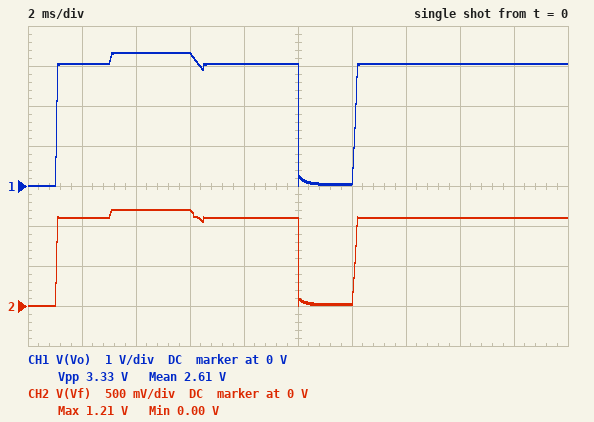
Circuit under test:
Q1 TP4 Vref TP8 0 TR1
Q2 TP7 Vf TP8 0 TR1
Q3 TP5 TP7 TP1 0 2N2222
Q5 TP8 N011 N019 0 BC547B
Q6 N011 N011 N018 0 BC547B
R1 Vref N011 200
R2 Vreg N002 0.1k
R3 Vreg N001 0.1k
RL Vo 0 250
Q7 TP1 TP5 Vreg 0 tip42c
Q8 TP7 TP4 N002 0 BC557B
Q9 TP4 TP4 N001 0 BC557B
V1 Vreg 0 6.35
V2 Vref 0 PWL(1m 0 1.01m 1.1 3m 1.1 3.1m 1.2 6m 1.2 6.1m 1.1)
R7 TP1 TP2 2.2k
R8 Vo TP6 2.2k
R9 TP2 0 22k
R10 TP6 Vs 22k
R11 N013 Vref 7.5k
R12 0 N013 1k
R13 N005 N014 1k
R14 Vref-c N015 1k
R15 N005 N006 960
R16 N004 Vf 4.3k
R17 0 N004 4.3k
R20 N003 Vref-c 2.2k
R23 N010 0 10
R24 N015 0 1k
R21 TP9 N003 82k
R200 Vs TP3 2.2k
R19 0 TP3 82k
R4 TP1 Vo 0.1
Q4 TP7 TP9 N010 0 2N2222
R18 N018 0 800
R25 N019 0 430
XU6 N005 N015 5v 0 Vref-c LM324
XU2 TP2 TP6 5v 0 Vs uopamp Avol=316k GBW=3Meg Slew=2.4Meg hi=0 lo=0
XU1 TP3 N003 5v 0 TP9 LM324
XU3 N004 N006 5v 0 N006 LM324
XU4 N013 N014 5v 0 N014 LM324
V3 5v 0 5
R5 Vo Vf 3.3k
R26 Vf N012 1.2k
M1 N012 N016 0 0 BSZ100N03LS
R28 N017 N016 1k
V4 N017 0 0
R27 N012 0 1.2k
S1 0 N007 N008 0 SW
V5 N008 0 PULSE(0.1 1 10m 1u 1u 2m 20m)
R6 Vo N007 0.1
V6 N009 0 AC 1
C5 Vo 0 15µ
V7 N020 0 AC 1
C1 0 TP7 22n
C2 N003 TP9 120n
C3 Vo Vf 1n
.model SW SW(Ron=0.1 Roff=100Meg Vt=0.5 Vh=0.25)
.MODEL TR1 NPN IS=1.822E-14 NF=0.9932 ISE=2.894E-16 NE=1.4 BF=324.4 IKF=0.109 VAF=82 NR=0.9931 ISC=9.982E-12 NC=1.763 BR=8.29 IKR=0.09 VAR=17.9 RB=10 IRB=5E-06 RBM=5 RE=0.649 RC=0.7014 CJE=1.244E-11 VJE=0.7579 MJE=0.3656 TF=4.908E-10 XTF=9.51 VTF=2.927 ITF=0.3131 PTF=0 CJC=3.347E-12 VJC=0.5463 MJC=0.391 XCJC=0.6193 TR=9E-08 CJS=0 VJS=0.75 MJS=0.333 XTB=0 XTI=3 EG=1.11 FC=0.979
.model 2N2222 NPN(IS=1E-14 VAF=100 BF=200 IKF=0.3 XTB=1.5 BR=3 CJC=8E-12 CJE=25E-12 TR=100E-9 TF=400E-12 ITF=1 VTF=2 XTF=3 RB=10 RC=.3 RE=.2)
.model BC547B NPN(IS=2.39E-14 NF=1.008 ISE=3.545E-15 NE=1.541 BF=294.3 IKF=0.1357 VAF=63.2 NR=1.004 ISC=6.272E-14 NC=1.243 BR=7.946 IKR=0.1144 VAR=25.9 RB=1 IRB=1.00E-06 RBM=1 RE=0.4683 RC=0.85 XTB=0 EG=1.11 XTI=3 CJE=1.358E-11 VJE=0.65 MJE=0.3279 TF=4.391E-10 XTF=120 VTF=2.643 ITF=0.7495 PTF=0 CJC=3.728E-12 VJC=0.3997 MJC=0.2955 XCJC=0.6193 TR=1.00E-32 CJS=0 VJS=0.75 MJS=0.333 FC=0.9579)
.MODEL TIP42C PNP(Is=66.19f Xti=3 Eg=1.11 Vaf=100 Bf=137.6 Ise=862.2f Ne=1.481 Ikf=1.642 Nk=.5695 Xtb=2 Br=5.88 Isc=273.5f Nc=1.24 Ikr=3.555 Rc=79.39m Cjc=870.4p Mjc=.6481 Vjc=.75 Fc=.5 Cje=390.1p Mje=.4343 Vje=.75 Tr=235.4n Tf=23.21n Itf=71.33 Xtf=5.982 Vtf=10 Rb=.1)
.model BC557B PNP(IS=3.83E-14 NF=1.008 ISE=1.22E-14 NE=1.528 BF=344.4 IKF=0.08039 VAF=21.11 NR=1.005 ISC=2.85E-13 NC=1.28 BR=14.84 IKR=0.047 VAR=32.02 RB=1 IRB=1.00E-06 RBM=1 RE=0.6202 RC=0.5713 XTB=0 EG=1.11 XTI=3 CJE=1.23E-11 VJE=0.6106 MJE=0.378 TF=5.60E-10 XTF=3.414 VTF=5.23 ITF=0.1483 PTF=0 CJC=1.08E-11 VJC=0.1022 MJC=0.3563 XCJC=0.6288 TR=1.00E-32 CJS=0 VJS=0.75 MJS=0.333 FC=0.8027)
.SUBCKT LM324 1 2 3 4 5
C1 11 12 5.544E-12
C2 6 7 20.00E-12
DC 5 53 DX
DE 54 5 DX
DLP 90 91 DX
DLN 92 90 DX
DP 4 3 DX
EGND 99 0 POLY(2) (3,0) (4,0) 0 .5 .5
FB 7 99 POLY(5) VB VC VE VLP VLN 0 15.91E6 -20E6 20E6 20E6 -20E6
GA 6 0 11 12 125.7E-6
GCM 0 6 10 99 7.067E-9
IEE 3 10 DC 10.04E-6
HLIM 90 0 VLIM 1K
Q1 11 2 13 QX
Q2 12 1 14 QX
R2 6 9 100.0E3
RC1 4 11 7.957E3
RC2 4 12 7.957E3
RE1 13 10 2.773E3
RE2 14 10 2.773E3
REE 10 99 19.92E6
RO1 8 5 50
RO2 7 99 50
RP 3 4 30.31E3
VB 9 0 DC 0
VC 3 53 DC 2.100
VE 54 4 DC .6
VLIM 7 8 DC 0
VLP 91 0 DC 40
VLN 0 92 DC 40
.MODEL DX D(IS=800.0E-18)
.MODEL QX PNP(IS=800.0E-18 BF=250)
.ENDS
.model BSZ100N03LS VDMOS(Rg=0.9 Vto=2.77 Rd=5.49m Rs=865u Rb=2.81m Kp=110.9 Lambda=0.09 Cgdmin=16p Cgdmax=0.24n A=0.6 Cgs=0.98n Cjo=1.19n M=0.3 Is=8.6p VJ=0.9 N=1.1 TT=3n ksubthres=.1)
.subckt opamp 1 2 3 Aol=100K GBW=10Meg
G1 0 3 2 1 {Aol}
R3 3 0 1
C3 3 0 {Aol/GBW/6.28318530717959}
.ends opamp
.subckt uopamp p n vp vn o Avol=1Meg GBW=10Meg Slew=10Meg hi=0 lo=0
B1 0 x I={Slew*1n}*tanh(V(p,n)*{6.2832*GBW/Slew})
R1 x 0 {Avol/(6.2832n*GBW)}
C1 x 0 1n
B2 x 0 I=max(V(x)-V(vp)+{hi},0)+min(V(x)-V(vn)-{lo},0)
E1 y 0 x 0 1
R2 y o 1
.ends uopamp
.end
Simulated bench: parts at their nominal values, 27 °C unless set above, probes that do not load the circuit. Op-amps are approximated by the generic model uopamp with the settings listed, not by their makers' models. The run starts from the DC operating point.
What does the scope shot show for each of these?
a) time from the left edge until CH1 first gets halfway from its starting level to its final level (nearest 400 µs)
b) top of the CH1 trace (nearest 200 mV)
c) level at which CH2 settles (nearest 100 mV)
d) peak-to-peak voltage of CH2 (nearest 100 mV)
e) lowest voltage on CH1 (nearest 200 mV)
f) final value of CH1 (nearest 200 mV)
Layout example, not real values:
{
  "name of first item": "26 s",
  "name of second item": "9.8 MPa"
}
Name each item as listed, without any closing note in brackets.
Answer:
{
  "time from the left edge until CH1 first gets halfway from its starting level to its final level": "1.2 ms",
  "top of the CH1 trace": "3.4 V",
  "level at which CH2 settles": "1.1 V",
  "peak-to-peak voltage of CH2": "1.2 V",
  "lowest voltage on CH1": "0 V",
  "final value of CH1": "3.0 V"
}
